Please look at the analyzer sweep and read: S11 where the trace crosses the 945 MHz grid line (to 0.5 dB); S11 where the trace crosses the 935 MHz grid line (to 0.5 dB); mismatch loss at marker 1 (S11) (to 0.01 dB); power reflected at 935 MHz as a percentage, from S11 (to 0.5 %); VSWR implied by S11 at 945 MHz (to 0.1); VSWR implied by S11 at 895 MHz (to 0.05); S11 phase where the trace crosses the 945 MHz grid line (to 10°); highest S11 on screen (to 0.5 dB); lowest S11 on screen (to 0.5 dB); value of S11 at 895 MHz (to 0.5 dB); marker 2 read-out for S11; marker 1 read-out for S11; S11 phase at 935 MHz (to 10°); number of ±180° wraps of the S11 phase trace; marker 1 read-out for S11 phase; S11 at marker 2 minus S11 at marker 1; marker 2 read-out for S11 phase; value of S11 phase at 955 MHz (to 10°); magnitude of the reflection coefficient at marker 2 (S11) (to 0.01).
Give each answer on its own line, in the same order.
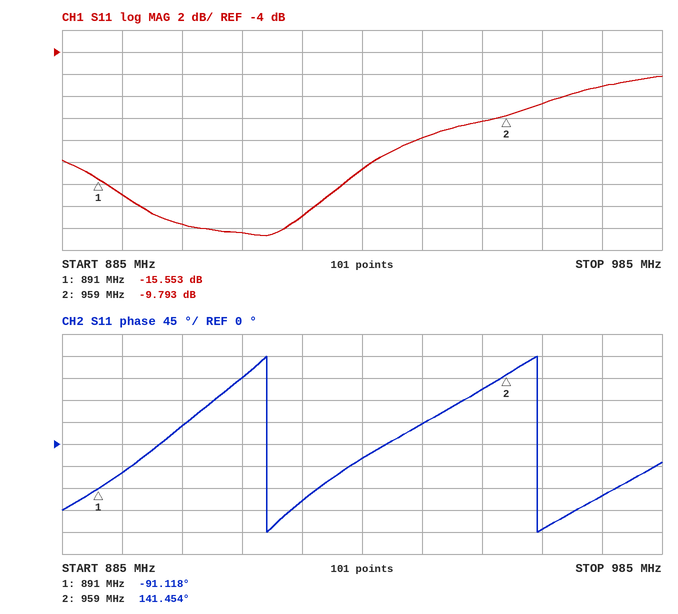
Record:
-12.0 dB
-14.5 dB
0.12 dB
3.5 %
1.7
1.35
40°
-6.0 dB
-20.5 dB
-17.0 dB
-9.793 dB
-15.553 dB
-30°
2
-91.118°
5.760 dB
141.454°
110°
0.32
